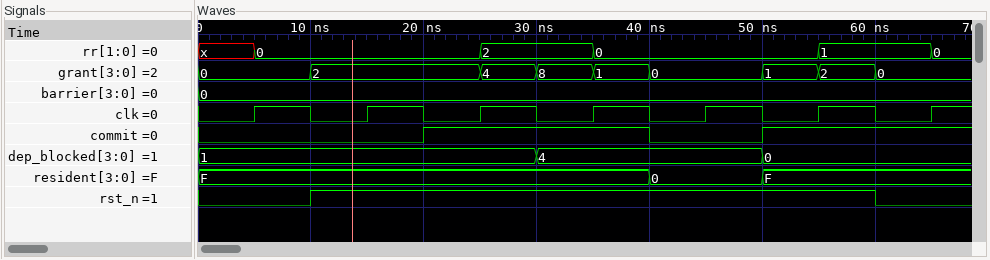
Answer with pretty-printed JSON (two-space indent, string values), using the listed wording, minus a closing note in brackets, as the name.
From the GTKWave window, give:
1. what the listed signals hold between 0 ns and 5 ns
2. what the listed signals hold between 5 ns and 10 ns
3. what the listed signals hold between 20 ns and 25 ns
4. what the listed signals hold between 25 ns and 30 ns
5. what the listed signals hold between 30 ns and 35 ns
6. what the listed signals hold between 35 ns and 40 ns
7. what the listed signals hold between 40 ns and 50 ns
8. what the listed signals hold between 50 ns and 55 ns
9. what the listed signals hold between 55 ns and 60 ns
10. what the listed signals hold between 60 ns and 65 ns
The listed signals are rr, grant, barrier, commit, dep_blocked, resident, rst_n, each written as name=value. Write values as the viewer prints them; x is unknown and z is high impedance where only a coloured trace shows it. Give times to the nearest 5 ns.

{
  "what the listed signals hold between 0 ns and 5 ns": "rr=x, grant=0, barrier=0, commit=0, dep_blocked=1, resident=F, rst_n=0",
  "what the listed signals hold between 5 ns and 10 ns": "rr=0, grant=0, barrier=0, commit=0, dep_blocked=1, resident=F, rst_n=0",
  "what the listed signals hold between 20 ns and 25 ns": "rr=0, grant=2, barrier=0, commit=1, dep_blocked=1, resident=F, rst_n=1",
  "what the listed signals hold between 25 ns and 30 ns": "rr=2, grant=4, barrier=0, commit=1, dep_blocked=1, resident=F, rst_n=1",
  "what the listed signals hold between 30 ns and 35 ns": "rr=2, grant=8, barrier=0, commit=1, dep_blocked=4, resident=F, rst_n=1",
  "what the listed signals hold between 35 ns and 40 ns": "rr=0, grant=1, barrier=0, commit=1, dep_blocked=4, resident=F, rst_n=1",
  "what the listed signals hold between 40 ns and 50 ns": "rr=0, grant=0, barrier=0, commit=0, dep_blocked=4, resident=0, rst_n=1",
  "what the listed signals hold between 50 ns and 55 ns": "rr=0, grant=1, barrier=0, commit=1, dep_blocked=0, resident=F, rst_n=1",
  "what the listed signals hold between 55 ns and 60 ns": "rr=1, grant=2, barrier=0, commit=1, dep_blocked=0, resident=F, rst_n=1",
  "what the listed signals hold between 60 ns and 65 ns": "rr=1, grant=0, barrier=0, commit=1, dep_blocked=0, resident=F, rst_n=0"
}
